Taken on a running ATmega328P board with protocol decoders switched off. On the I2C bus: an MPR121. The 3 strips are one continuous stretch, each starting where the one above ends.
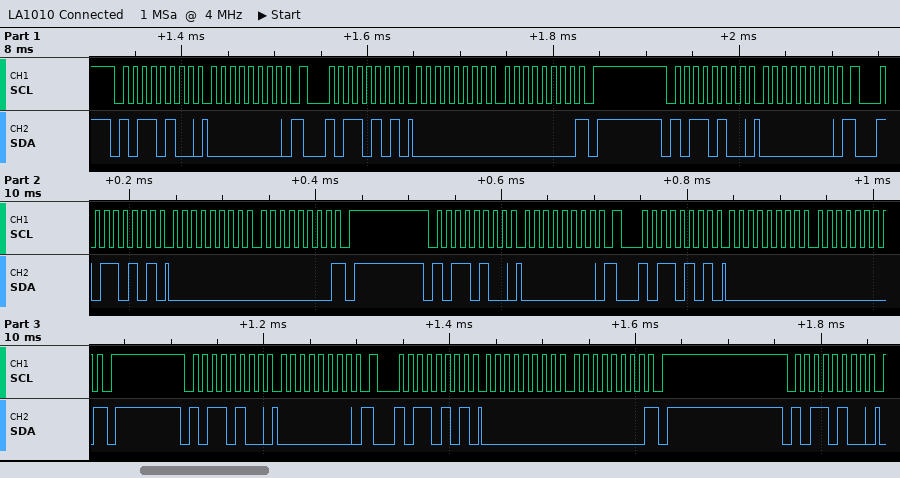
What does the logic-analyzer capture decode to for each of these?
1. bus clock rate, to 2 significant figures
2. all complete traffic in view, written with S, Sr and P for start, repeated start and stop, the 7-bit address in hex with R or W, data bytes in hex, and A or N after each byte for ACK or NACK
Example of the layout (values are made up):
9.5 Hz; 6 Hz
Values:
100 kHz; S 5AW A 00 A Sr 5AR A 00 A 00 N P S 5AW A 00 A Sr 5AR A 00 A 00 N P S 5AW A 00 A Sr 5AR A 00 A 00 N P S 5AW A 00 A Sr 5AR A 00 A 00 N P S 5AW A
